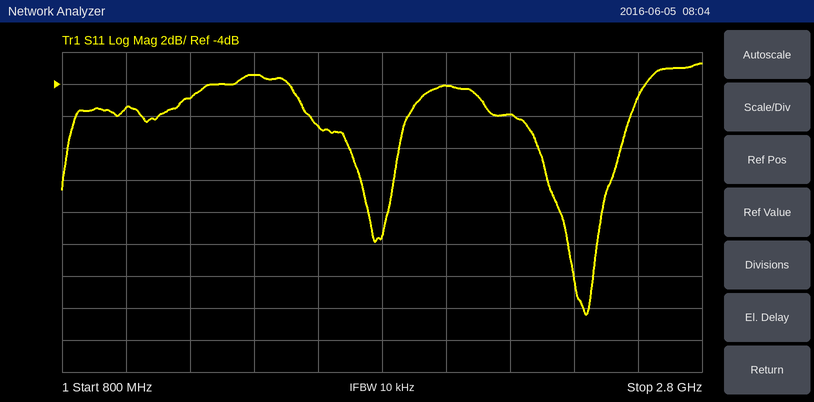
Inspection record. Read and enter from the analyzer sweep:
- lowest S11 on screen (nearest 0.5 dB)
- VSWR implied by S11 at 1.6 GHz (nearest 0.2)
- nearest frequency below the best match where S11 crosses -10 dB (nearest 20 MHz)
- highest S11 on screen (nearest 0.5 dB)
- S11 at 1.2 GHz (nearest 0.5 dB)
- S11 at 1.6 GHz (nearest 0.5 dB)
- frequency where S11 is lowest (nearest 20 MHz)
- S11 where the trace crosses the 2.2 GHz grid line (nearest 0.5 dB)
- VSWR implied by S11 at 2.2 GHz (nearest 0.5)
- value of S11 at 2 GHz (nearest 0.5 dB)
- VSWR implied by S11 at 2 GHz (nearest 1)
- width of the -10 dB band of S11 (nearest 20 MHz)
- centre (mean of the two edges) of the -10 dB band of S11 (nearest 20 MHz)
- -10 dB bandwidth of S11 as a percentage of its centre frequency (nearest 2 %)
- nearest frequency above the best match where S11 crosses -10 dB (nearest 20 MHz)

-18.5 dB
2.8
2.32 GHz
-2.5 dB
-5.0 dB
-6.5 dB
2.44 GHz
-6.0 dB
3.0
-4.0 dB
4
200 MHz
2.42 GHz
8 %
2.52 GHz
